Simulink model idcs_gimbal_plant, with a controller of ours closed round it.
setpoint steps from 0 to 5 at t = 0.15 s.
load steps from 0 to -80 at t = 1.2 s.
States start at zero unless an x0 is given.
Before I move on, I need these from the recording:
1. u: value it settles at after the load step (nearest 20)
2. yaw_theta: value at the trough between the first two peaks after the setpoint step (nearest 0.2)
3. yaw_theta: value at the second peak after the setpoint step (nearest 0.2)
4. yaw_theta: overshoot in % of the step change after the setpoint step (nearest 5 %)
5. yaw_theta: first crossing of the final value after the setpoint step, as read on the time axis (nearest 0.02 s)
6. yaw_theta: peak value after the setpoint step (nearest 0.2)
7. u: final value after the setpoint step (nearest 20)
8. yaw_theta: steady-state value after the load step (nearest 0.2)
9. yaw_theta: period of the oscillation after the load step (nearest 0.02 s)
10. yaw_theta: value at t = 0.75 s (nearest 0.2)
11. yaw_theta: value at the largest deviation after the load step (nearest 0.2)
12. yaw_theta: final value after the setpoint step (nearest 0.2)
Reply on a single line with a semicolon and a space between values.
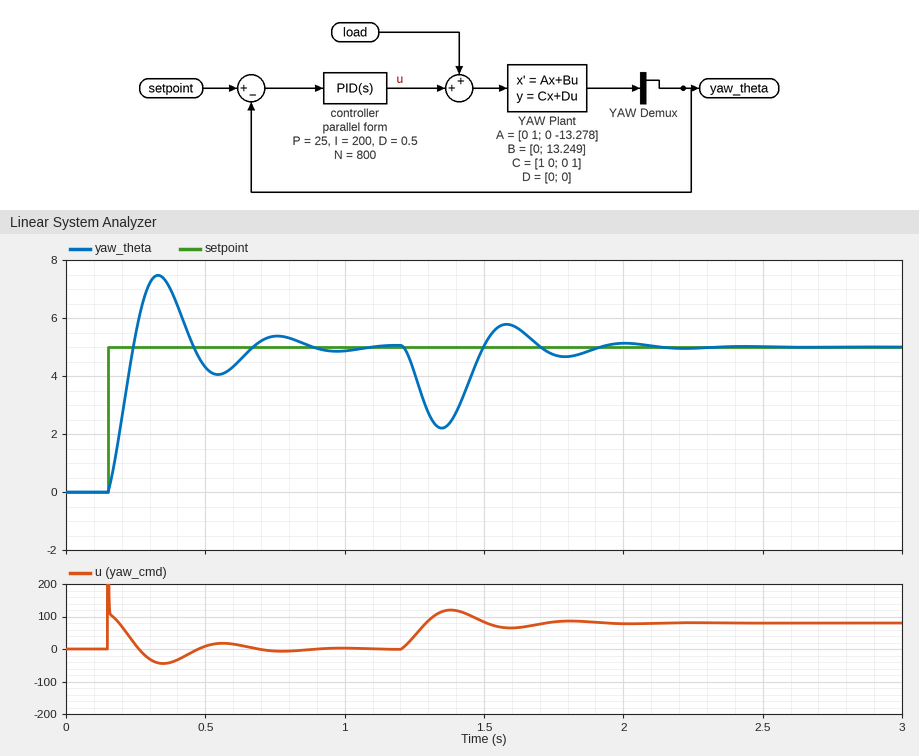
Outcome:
80; 4.0; 5.4; 50 %; 0.24 s; 7.4; 0; 5.0; 0.44 s; 5.4; 2.2; 5.0
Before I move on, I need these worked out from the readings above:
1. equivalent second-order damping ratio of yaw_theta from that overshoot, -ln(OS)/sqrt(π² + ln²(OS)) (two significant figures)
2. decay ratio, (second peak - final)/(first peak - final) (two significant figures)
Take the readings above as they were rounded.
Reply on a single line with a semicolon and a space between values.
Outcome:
0.22; 0.17
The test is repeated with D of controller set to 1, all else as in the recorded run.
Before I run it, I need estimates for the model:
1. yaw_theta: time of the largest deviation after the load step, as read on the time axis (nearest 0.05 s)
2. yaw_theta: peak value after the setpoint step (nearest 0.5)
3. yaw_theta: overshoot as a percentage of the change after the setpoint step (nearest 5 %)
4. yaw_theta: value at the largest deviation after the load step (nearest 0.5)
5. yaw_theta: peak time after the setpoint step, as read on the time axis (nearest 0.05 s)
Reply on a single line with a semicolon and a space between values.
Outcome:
1.35 s; 6.5; 35 %; 2.5; 0.35 s
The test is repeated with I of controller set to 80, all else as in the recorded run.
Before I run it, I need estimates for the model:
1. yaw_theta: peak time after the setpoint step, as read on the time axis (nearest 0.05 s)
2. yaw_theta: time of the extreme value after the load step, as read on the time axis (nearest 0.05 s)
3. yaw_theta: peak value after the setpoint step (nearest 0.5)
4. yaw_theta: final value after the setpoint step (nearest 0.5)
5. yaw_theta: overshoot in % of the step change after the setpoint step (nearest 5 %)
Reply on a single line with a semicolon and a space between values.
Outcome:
0.35 s; 1.35 s; 6.5; 5.0; 30 %
